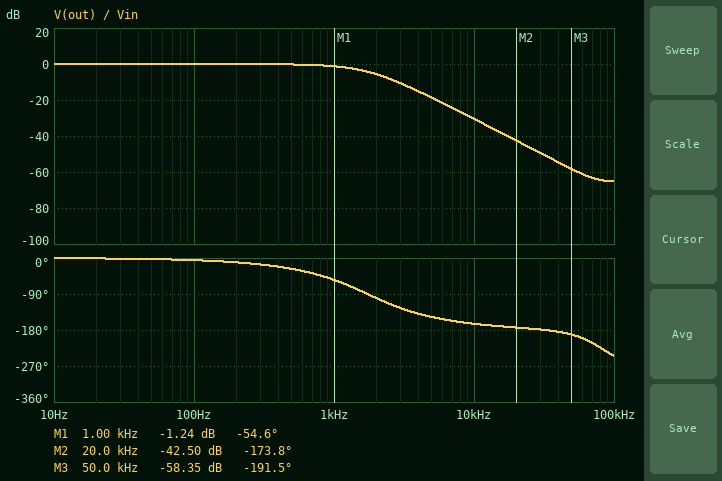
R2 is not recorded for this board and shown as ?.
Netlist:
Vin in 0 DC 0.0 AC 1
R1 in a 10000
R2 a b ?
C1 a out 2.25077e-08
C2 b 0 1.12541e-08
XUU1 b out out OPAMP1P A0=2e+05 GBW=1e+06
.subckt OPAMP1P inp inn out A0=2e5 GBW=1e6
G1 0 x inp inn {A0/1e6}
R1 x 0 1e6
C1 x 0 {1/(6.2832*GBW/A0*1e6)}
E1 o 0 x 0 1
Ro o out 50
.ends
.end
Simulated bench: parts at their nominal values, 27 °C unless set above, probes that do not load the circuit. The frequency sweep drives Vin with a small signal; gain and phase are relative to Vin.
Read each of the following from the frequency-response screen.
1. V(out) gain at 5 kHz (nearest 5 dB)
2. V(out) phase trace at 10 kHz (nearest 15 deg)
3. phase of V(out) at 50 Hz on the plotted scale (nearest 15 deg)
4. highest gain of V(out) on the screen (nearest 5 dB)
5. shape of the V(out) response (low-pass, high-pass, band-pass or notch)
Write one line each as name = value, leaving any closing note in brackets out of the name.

V(out) gain at 5 kHz = -20 dB
V(out) phase trace at 10 kHz = -165 deg
phase of V(out) at 50 Hz on the plotted scale = 0 deg
highest gain of V(out) on the screen = 0 dB
shape of the V(out) response = low-pass
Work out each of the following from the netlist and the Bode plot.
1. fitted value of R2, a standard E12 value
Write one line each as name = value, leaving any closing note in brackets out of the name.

fitted value of R2, a standard E12 value = 3.3 kΩ
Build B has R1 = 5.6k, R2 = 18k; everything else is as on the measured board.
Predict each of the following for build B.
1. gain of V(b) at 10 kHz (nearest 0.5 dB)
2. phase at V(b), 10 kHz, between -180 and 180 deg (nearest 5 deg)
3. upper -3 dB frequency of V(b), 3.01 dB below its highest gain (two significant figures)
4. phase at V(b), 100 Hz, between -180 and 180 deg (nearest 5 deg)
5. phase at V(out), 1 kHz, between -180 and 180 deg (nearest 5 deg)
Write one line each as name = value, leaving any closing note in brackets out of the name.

gain of V(b) at 10 kHz = -40.0 dB
phase at V(b), 10 kHz, between -180 and 180 deg = -170 deg
upper -3 dB frequency of V(b), 3.01 dB below its highest gain = 830 Hz
phase at V(b), 100 Hz, between -180 and 180 deg = -10 deg
phase at V(out), 1 kHz, between -180 and 180 deg = -90 deg
